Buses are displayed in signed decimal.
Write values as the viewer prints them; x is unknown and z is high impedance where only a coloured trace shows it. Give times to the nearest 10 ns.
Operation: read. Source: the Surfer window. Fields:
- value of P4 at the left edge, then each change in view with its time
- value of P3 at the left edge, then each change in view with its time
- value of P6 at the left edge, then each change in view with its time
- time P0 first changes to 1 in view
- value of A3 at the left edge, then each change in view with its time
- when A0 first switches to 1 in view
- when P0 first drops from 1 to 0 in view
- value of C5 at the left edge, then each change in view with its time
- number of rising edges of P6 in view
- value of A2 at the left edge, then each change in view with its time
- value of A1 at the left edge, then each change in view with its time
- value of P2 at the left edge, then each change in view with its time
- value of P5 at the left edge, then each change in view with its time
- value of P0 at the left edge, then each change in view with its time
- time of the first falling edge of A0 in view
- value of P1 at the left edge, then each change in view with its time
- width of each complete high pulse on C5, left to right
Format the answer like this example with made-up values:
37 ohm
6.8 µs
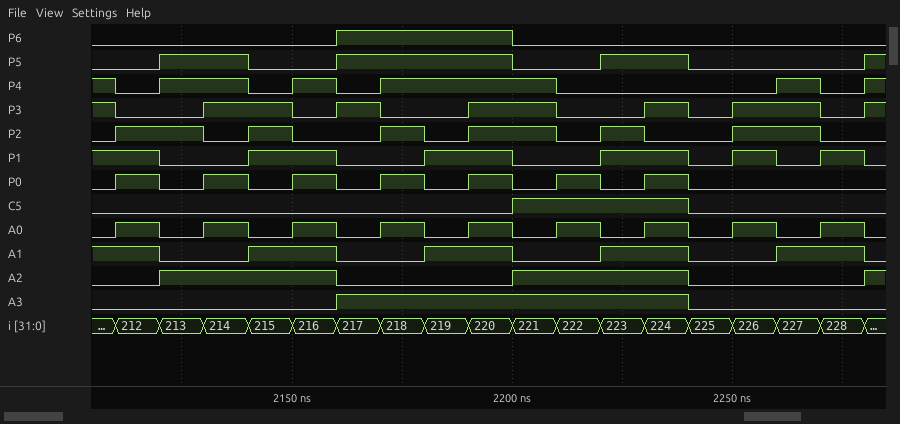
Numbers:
1, 0 at 2110 ns, 1 at 2120 ns, 0 at 2140 ns, 1 at 2150 ns, 0 at 2160 ns, 1 at 2170 ns, 0 at 2210 ns, 1 at 2260 ns, 0 at 2270 ns, 1 at 2280 ns
1, 0 at 2110 ns, 1 at 2130 ns, 0 at 2150 ns, 1 at 2160 ns, 0 at 2170 ns, 1 at 2190 ns, 0 at 2210 ns, 1 at 2230 ns, 0 at 2240 ns, 1 at 2250 ns, 0 at 2270 ns, 1 at 2280 ns
0, 1 at 2160 ns, 0 at 2200 ns
2110 ns
0, 1 at 2160 ns, 0 at 2240 ns
2110 ns
2120 ns
0, 1 at 2200 ns, 0 at 2240 ns
1
0, 1 at 2120 ns, 0 at 2160 ns, 1 at 2200 ns, 0 at 2240 ns, 1 at 2280 ns
1, 0 at 2120 ns, 1 at 2140 ns, 0 at 2160 ns, 1 at 2180 ns, 0 at 2200 ns, 1 at 2220 ns, 0 at 2240 ns, 1 at 2260 ns, 0 at 2280 ns
0, 1 at 2110 ns, 0 at 2130 ns, 1 at 2140 ns, 0 at 2150 ns, 1 at 2170 ns, 0 at 2180 ns, 1 at 2190 ns, 0 at 2210 ns, 1 at 2220 ns, 0 at 2230 ns, 1 at 2250 ns, 0 at 2270 ns
0, 1 at 2120 ns, 0 at 2140 ns, 1 at 2160 ns, 0 at 2200 ns, 1 at 2220 ns, 0 at 2240 ns, 1 at 2280 ns
0, 1 at 2110 ns, 0 at 2120 ns, 1 at 2130 ns, 0 at 2140 ns, 1 at 2150 ns, 0 at 2160 ns, 1 at 2170 ns, 0 at 2180 ns, 1 at 2190 ns, 0 at 2200 ns, 1 at 2210 ns, 0 at 2220 ns, 1 at 2230 ns, 0 at 2240 ns
2120 ns
1, 0 at 2120 ns, 1 at 2140 ns, 0 at 2160 ns, 1 at 2180 ns, 0 at 2200 ns, 1 at 2220 ns, 0 at 2240 ns, 1 at 2250 ns, 0 at 2260 ns, 1 at 2270 ns, 0 at 2280 ns
40 ns
